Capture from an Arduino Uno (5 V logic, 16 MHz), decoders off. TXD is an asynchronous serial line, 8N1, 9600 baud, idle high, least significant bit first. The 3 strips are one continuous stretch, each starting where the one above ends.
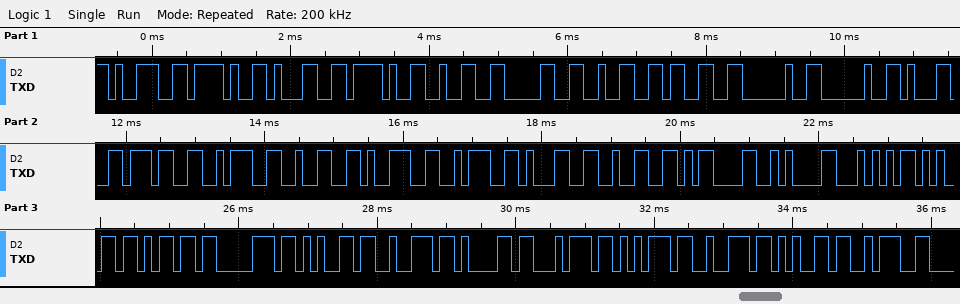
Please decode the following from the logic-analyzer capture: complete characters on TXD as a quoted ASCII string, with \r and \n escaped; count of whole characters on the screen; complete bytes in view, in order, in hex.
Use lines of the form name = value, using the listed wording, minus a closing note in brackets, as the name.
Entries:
complete characters on TXD as a quoted ASCII string, with \r and \n escaped = "9/1/2023  17:29:12\r\nTemperature:"
count of whole characters on the screen = 32
complete bytes in view, in order, in hex = 39 2F 31 2F 32 30 32 33 20 20 31 37 3A 32 39 3A 31 32 0D 0A 54 65 6D 70 65 72 61 74 75 72 65 3A
